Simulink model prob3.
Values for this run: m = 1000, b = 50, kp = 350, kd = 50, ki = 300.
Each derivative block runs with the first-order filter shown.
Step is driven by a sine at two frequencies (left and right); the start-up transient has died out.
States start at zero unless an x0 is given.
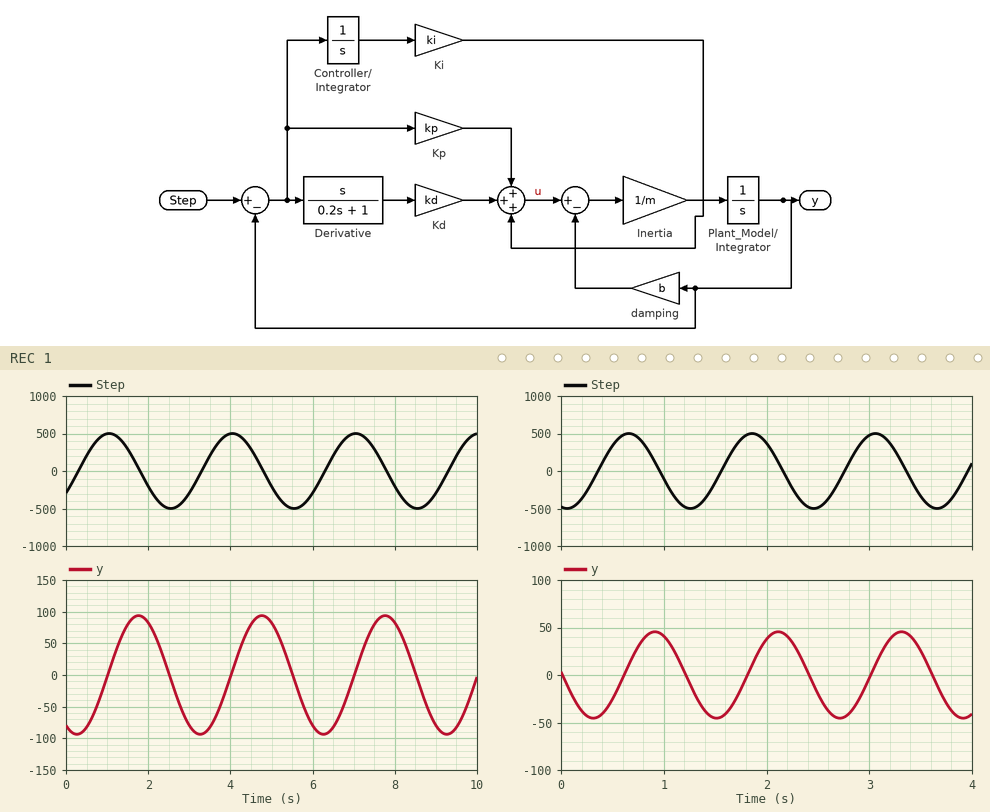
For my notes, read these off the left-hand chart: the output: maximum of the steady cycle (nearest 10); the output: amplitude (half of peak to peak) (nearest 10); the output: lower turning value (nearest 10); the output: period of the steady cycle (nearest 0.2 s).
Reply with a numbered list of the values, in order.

1. 90
2. 90
3. -90
4. 3.0 s
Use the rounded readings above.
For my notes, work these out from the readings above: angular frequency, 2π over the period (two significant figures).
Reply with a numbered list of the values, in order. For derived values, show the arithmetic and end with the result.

1. 2π / 3 = 2.1 rad/s
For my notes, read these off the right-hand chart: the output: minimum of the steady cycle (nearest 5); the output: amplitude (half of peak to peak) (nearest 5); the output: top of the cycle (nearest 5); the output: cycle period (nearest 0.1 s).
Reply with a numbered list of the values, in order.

1. -45
2. 45
3. 45
4. 1.2 s
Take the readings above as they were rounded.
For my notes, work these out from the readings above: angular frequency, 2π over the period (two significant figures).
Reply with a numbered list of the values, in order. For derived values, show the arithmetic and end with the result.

1. 2π / 1.2 = 5.2 rad/s
